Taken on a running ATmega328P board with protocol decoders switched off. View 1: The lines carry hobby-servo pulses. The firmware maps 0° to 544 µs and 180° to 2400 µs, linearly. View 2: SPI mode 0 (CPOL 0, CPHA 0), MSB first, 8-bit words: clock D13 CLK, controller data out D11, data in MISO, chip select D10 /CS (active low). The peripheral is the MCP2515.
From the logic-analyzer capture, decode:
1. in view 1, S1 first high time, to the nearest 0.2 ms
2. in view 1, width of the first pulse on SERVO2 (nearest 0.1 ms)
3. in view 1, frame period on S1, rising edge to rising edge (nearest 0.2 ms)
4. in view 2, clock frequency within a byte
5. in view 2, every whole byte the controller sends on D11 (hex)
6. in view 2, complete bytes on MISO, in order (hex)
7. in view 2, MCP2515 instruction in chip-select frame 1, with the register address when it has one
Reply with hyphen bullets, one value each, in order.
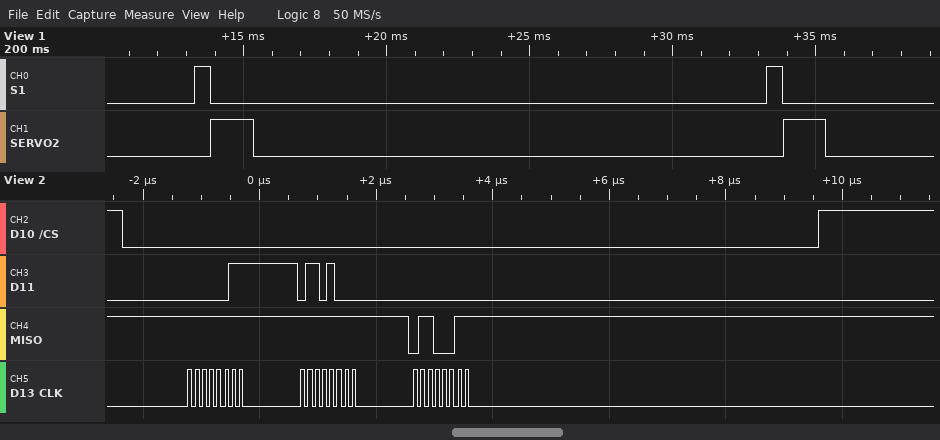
- 0.6 ms
- 1.5 ms
- 20.0 ms
- 8 MHz
- 03 68 00
- FF FF 63
- READ 0x68
